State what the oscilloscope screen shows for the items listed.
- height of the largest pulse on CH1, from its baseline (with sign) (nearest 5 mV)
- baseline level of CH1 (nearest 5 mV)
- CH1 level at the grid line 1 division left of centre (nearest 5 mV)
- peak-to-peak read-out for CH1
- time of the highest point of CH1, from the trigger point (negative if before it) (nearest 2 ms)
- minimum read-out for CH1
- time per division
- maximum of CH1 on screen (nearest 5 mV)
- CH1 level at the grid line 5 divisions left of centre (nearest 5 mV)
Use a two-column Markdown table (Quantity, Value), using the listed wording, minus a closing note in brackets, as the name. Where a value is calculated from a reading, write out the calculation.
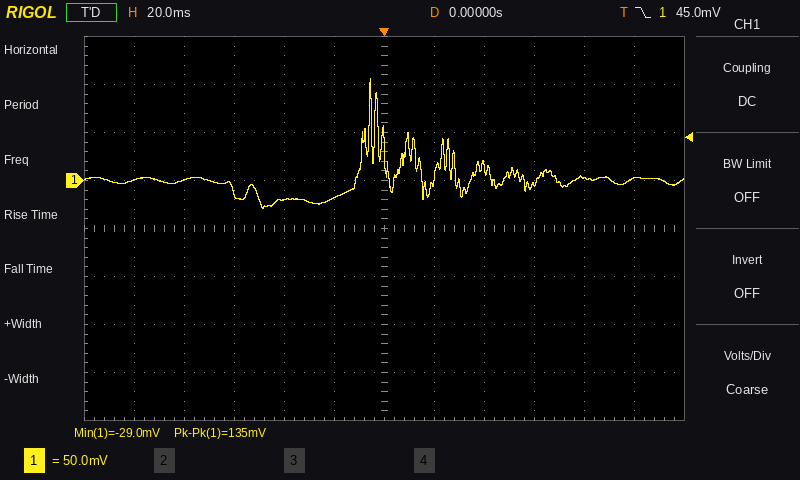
| Quantity | Value |
|---|---|
| height of the largest pulse on CH1, from its baseline (with sign) | 105 mV − (0 mV) = +105 mV |
| baseline level of CH1 | 0 mV |
| CH1 level at the grid line 1 division left of centre | -20 mV |
| peak-to-peak read-out for CH1 | 135 mV |
| time of the highest point of CH1, from the trigger point (negative if before it) | -6 ms |
| minimum read-out for CH1 | -29.0 mV |
| time per division | 20 ms |
| maximum of CH1 on screen | 105 mV |
| CH1 level at the grid line 5 divisions left of centre | 0 mV |
